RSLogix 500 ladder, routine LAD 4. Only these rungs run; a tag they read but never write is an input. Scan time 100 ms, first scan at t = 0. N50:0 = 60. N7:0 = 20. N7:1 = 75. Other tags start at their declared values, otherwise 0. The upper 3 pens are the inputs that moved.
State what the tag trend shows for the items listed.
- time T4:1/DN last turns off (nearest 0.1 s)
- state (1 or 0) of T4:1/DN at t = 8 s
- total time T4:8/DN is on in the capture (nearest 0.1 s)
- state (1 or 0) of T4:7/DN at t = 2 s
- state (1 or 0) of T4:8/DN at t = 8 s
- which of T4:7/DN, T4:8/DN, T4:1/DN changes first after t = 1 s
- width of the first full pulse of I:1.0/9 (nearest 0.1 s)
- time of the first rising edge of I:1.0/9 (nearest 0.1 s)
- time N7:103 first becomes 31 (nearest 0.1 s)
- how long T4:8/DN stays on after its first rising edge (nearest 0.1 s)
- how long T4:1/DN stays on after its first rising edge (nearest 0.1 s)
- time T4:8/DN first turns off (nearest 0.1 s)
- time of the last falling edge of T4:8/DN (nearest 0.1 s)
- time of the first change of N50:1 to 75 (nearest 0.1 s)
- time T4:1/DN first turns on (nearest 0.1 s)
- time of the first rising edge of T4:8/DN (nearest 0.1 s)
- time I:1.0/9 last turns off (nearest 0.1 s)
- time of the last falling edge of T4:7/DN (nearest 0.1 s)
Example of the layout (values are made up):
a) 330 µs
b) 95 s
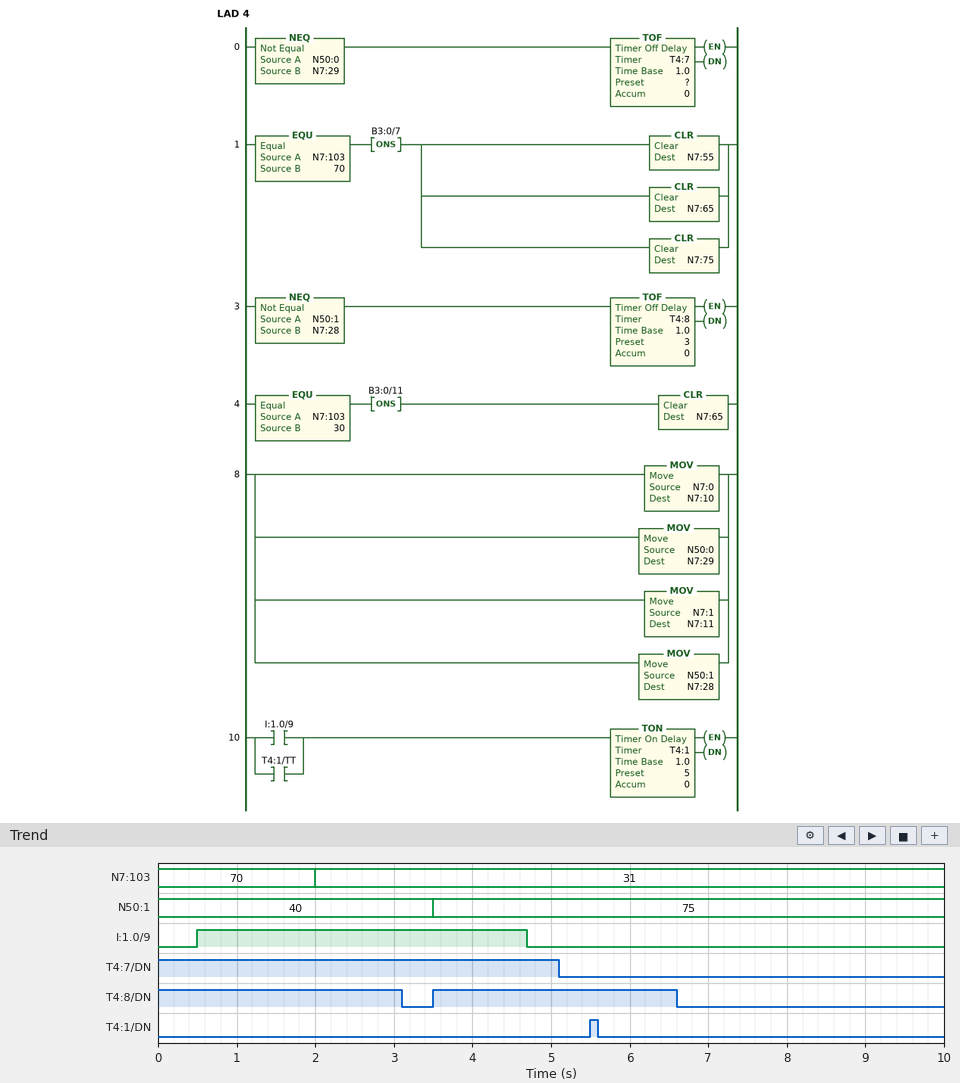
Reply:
a) 5.6 s
b) 0
c) 6.2 s
d) 1
e) 0
f) T4:8/DN
g) 4.2 s
h) 0.5 s
i) 2.0 s
j) 3.1 s
k) 0.1 s
l) 3.1 s
m) 6.6 s
n) 3.5 s
o) 5.5 s
p) 3.5 s
q) 4.7 s
r) 5.1 s
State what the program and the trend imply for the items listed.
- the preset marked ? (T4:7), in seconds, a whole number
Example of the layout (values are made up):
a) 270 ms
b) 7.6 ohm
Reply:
a) 5 s
